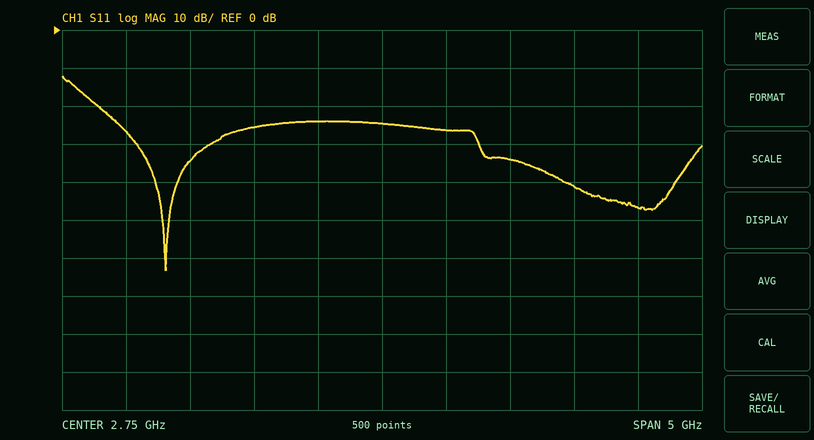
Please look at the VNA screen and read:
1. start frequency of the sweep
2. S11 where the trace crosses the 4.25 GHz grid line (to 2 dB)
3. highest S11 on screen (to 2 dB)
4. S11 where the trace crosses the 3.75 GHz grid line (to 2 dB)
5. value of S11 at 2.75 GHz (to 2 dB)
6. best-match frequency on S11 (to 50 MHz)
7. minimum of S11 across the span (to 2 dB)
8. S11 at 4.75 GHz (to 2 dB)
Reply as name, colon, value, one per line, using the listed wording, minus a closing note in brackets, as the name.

start frequency of the sweep: 250 MHz
S11 where the trace crosses the 4.25 GHz grid line: -42 dB
highest S11 on screen: -12 dB
S11 where the trace crosses the 3.75 GHz grid line: -34 dB
value of S11 at 2.75 GHz: -24 dB
best-match frequency on S11: 1.05 GHz
minimum of S11 across the span: -64 dB
S11 at 4.75 GHz: -46 dB
